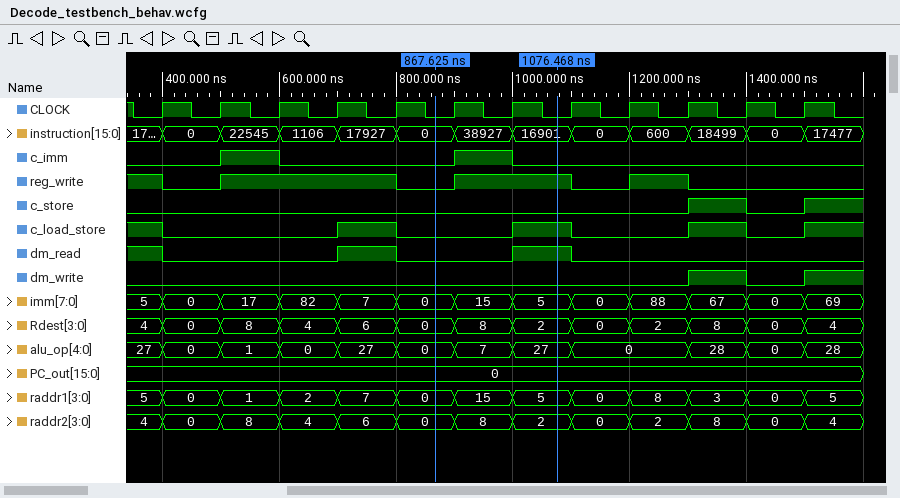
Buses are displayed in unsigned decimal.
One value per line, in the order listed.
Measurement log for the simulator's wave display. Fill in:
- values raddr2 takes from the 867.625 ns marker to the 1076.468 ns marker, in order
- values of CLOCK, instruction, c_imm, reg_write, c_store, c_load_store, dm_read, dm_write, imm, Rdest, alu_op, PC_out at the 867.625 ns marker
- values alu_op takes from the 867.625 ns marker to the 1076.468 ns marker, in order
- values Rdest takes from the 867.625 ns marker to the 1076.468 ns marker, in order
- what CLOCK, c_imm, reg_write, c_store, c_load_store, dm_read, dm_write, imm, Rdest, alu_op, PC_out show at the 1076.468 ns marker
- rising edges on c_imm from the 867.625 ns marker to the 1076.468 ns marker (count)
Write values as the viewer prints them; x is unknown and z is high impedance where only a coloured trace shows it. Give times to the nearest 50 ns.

0, 8, 2
CLOCK=0, instruction=0, c_imm=0, reg_write=0, c_store=0, c_load_store=0, dm_read=0, dm_write=0, imm=0, Rdest=0, alu_op=0, PC_out=0
0, 7, 27
0, 8, 2
CLOCK=0, c_imm=0, reg_write=1, c_store=0, c_load_store=1, dm_read=1, dm_write=0, imm=5, Rdest=2, alu_op=27, PC_out=0
1
